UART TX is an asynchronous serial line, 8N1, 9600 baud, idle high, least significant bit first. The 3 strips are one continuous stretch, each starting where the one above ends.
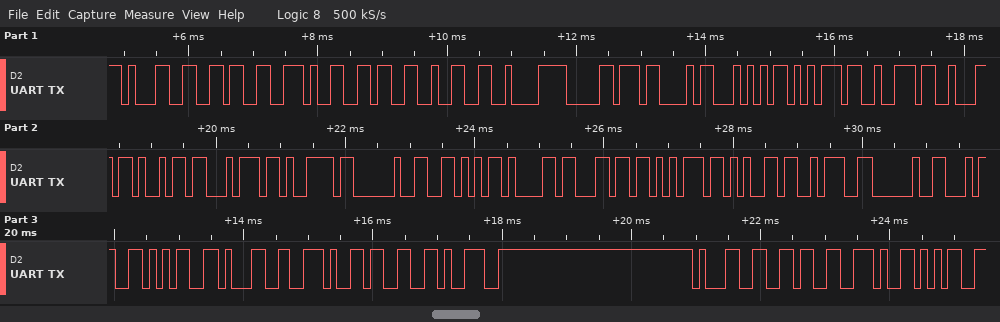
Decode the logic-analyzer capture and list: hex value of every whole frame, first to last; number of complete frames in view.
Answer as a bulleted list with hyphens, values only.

- 31 36 2E 36 32 C2 B0 43 54 75 72 62 69 74 79 20 56 61 6C 75 65 3A 20 34 35 31 2E 33 39 31 36 2E 35
- 33
